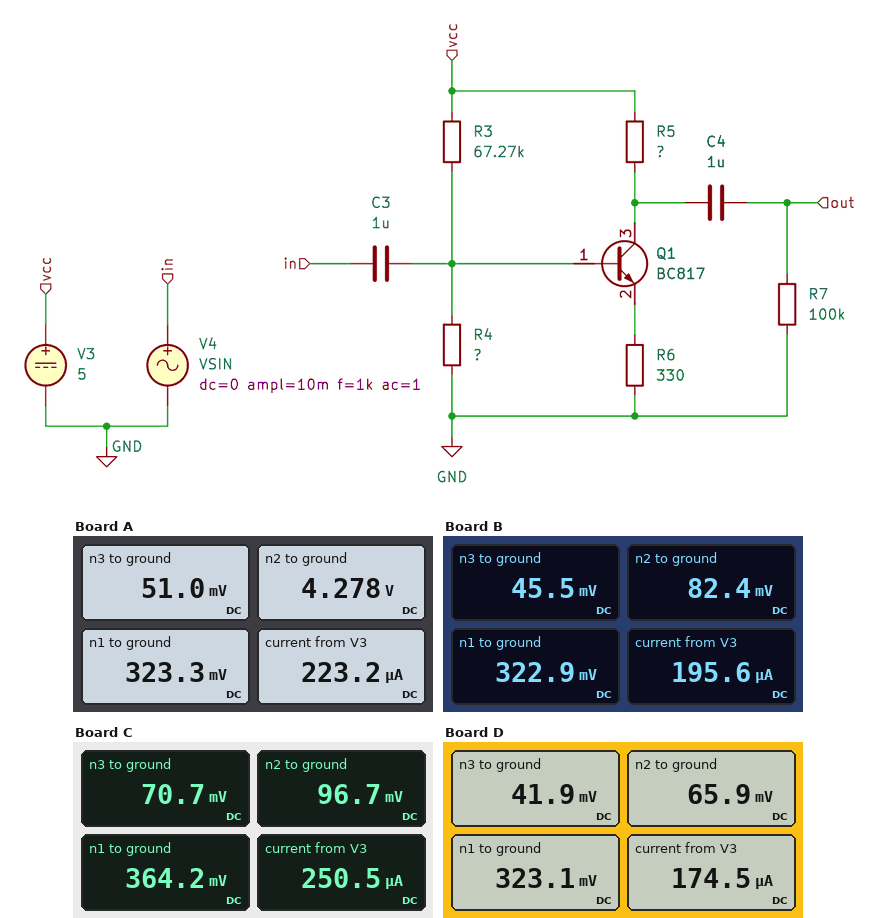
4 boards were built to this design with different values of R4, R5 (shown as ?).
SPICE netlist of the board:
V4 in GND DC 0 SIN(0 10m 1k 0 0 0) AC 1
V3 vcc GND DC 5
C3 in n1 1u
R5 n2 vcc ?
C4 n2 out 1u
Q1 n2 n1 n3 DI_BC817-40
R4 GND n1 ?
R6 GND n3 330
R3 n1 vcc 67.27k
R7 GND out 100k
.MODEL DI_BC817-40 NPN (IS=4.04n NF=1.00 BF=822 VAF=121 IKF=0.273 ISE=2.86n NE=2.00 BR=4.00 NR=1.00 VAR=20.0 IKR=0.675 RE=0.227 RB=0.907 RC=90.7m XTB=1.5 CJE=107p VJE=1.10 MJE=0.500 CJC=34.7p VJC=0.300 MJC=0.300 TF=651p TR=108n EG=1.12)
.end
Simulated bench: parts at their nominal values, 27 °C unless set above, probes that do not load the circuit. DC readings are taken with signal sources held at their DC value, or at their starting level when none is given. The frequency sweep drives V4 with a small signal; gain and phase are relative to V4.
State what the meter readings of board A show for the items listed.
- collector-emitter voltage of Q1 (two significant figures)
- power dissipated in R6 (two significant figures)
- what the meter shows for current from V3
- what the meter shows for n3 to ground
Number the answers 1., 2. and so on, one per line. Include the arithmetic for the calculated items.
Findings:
1. 4.278 V - 51 mV = 4.2 V
2. (51 mV)^2 / 330 Ω = 7.9 µW
3. 223.2 µA
4. 51.0 mV
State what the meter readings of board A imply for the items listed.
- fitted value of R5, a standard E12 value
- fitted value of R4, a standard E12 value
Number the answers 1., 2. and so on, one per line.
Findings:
1. 4.7 kΩ
2. 4.7 kΩ
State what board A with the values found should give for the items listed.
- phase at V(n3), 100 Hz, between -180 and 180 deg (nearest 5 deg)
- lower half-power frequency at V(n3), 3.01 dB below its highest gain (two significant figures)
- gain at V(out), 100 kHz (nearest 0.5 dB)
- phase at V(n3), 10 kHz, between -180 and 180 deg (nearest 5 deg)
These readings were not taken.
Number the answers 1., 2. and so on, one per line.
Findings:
1. 20 deg
2. 3.9 MHz
3. 19.0 dB
4. 0 deg
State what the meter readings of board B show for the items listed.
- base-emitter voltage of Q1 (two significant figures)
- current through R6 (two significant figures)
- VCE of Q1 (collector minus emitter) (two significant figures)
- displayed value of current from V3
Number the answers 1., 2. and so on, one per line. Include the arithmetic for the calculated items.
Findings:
1. 322.9 mV - 45.5 mV = 280 mV
2. (45.5 mV) / 330 Ω = 140 µA
3. 82.4 mV - 45.5 mV = 37 mV
4. 195.6 µA
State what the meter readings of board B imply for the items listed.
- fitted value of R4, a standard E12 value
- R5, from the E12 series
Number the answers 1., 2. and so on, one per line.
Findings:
1. 5.6 kΩ
2. 39 kΩ
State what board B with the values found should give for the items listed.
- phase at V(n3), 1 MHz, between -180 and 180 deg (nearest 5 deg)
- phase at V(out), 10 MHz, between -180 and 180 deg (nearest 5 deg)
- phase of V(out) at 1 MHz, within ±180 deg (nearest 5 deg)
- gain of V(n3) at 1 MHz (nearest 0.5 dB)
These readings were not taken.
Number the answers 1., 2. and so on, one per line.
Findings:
1. 20 deg
2. 5 deg
3. 65 deg
4. -3.5 dB
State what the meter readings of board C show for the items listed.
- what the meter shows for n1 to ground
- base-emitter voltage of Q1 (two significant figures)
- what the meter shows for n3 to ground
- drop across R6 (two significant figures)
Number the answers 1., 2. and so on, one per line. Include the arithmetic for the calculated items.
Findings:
1. 364.2 mV
2. 364.2 mV - 70.7 mV = 290 mV
3. 70.7 mV
4. 70.7 mV = 71 mV
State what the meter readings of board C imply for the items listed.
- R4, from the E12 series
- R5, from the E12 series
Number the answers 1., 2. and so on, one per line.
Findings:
1. 10 kΩ
2. 27 kΩ
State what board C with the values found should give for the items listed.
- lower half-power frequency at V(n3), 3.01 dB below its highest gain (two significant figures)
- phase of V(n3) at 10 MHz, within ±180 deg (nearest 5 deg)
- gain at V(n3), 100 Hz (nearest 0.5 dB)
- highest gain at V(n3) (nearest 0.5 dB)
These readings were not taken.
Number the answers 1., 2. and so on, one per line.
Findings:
1. 680 kHz
2. 5 deg
3. -15.0 dB
4. 0 dB
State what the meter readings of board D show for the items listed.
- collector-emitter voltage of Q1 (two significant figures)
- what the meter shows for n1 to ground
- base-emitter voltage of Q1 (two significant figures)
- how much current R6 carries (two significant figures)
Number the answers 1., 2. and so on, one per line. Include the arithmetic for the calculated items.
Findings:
1. 65.9 mV - 41.9 mV = 24 mV
2. 323.1 mV
3. 323.1 mV - 41.9 mV = 280 mV
4. (41.9 mV) / 330 Ω = 130 µA
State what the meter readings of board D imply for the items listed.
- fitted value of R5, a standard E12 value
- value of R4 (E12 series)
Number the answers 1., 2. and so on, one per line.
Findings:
1. 47 kΩ
2. 6.8 kΩ
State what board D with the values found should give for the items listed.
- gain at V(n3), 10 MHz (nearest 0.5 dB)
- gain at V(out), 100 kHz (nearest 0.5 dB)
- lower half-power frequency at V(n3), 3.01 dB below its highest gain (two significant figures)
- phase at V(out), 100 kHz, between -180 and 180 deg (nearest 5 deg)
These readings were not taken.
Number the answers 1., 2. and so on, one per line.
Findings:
1. -1.5 dB
2. -9.5 dB
3. 1.3 MHz
4. 140 deg
